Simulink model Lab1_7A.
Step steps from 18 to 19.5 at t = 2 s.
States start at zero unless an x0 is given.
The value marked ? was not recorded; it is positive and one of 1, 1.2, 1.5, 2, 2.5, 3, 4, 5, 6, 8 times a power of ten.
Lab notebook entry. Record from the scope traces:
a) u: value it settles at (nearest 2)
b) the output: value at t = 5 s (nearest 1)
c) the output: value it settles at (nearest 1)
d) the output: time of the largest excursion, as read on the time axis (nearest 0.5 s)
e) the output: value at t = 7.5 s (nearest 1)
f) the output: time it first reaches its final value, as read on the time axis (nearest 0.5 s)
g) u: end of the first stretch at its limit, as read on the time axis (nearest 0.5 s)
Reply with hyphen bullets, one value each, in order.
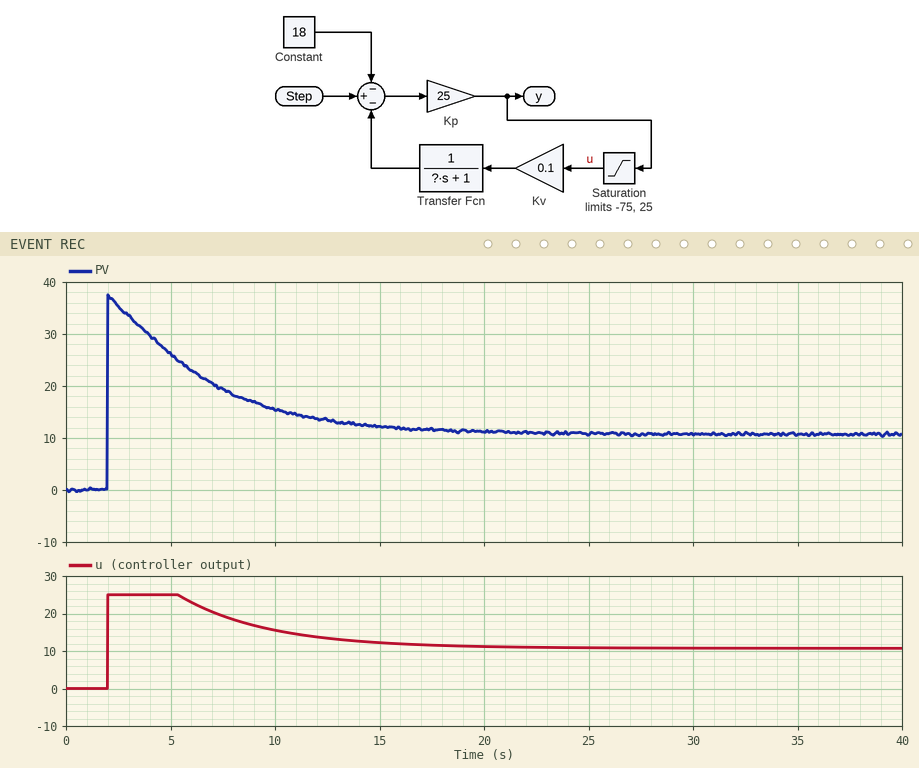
- 10
- 26
- 11
- 2.0 s
- 19
- 2.0 s
- 5.5 s
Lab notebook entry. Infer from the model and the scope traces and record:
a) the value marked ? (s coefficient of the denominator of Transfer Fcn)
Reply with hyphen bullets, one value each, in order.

- 15
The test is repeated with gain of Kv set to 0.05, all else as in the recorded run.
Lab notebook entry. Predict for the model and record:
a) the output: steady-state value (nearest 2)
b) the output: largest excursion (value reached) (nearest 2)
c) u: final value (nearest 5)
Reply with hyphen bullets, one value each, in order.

- 16
- 38
- 15
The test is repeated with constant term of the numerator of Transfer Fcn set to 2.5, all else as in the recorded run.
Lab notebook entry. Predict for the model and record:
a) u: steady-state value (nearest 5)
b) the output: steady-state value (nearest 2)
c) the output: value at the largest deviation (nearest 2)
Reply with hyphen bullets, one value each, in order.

- 5
- 6
- 38
